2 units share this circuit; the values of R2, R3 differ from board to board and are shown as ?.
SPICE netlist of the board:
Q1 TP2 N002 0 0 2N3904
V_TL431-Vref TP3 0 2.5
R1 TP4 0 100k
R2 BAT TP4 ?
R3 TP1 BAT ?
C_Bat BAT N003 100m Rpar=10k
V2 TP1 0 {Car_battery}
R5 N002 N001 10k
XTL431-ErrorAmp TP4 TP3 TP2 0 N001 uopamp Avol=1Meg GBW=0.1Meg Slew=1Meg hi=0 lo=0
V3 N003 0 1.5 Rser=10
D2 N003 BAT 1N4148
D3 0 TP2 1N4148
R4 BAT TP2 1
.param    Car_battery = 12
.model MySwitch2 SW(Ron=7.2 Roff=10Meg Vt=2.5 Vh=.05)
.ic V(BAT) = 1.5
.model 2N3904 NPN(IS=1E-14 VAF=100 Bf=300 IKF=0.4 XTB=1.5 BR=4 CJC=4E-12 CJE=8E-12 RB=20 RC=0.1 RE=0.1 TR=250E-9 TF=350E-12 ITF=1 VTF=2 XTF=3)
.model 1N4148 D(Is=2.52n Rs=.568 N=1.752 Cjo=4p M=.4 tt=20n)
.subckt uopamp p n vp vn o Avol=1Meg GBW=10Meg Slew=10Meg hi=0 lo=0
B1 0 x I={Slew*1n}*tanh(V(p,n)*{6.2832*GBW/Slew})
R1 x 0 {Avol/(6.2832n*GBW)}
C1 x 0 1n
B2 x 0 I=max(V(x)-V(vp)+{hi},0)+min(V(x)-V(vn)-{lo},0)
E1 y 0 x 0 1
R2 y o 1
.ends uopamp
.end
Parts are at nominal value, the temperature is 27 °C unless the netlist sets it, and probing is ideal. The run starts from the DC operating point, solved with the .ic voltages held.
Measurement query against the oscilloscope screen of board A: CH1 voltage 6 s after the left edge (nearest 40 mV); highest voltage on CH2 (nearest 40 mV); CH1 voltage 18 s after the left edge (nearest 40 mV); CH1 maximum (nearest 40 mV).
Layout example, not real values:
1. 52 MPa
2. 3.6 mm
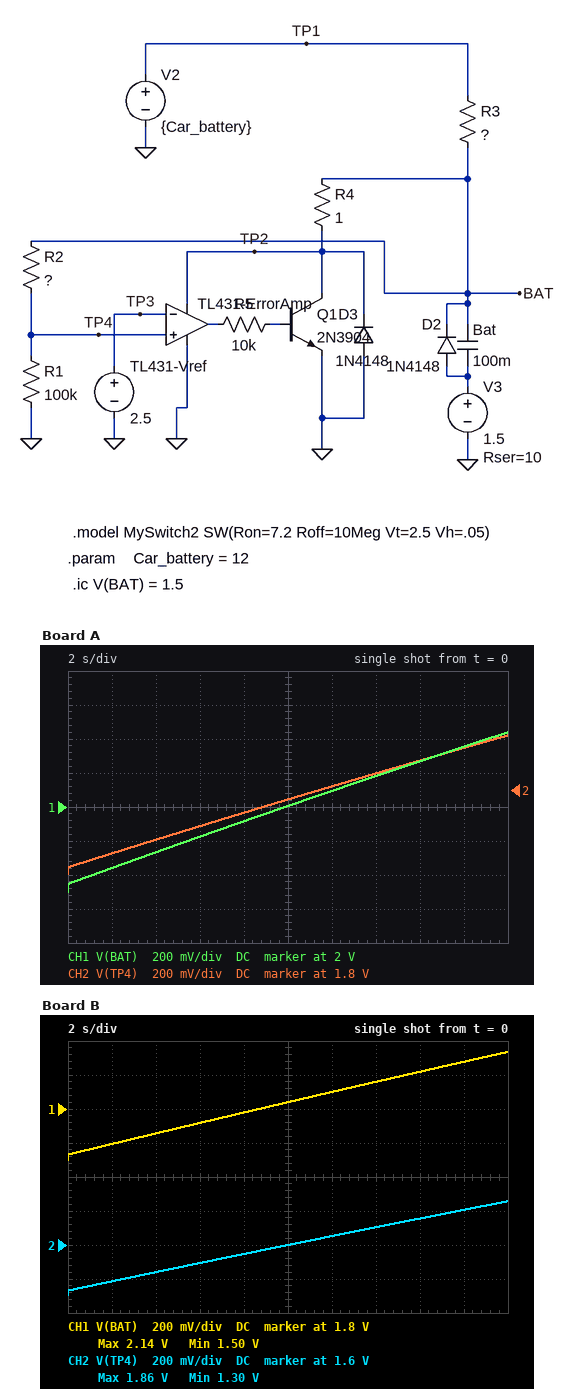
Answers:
1. 1.84 V
2. 2.12 V
3. 2.36 V
4. 2.44 V
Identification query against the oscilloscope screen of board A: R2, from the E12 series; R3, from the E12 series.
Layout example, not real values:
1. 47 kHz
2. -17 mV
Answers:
1. 15 kΩ
2. 2.2 kΩ
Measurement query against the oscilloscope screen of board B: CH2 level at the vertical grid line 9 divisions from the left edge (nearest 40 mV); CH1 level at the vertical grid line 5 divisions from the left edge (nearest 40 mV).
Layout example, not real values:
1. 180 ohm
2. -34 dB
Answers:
1. 1.80 V
2. 1.84 V
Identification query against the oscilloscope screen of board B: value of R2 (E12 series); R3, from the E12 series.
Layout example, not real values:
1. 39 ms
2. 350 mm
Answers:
1. 15 kΩ
2. 3.3 kΩ
